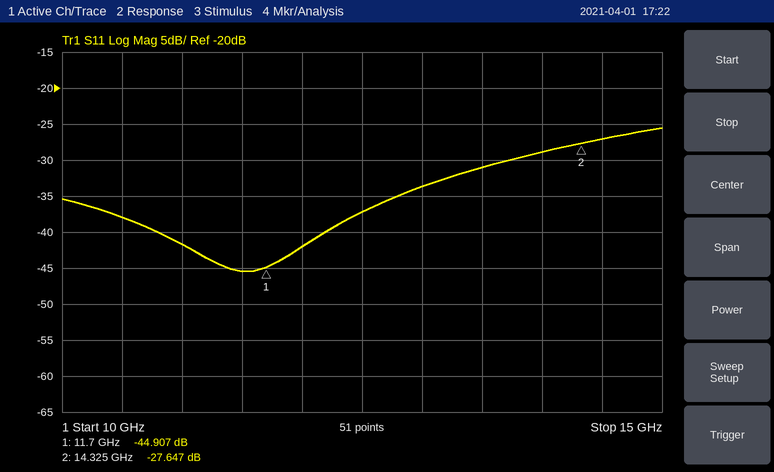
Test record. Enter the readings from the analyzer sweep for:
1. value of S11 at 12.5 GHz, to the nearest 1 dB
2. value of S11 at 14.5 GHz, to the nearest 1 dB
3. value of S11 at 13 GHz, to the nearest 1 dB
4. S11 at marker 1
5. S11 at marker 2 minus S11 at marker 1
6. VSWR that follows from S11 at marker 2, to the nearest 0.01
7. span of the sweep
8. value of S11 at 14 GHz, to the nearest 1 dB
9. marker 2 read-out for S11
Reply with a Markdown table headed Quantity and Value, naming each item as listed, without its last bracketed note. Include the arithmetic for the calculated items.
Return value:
| Quantity | Value |
|---|---|
| value of S11 at 12.5 GHz, to the nearest 1 dB | -37 dB |
| value of S11 at 14.5 GHz, to the nearest 1 dB | -27 dB |
| value of S11 at 13 GHz, to the nearest 1 dB | -34 dB |
| S11 at marker 1 | -44.907 dB |
| S11 at marker 2 minus S11 at marker 1 | -27.647 − (-44.907) = 17.260 dB |
| VSWR that follows from S11 at marker 2, to the nearest 0.01 | (1 + 0.0415)/(1 − 0.0415) ≈ 1.09 |
| span of the sweep | 5 GHz |
| value of S11 at 14 GHz, to the nearest 1 dB | -29 dB |
| marker 2 read-out for S11 | -27.647 dB |
